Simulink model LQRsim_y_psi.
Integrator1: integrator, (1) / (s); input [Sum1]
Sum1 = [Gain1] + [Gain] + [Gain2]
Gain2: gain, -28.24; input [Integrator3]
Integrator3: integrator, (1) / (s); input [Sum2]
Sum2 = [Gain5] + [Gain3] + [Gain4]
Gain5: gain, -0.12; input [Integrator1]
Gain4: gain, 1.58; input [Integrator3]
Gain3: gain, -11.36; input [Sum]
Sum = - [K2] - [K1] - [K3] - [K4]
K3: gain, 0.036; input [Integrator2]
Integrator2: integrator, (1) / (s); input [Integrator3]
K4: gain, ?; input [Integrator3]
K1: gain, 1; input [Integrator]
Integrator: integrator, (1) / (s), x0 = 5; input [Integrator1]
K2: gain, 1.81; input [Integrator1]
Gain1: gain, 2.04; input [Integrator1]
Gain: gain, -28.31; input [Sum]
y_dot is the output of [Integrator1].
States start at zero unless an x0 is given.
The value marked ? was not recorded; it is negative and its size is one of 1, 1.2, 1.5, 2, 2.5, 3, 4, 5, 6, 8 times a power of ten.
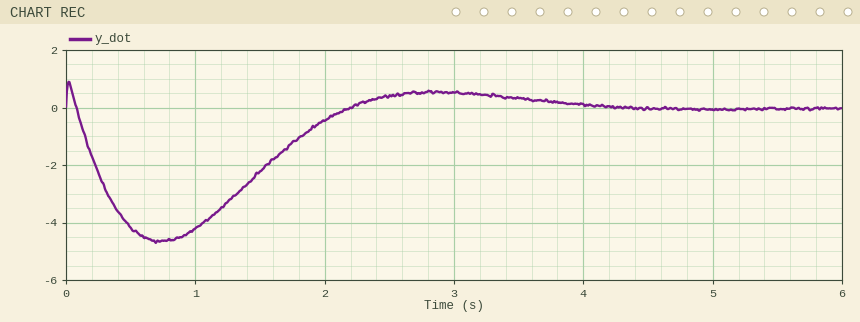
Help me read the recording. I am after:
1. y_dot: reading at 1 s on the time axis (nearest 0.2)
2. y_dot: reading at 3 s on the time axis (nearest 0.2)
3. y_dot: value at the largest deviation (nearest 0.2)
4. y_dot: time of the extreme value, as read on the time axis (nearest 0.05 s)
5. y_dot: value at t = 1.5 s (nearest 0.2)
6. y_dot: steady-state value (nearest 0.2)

-4.2
0.6
-4.6
0.75 s
-2.2
0.0
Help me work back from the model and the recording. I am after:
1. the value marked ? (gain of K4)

-15
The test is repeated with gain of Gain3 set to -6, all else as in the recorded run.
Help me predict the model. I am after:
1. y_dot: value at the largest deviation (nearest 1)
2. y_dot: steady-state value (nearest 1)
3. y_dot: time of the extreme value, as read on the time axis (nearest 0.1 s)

-6
0
0.6 s
